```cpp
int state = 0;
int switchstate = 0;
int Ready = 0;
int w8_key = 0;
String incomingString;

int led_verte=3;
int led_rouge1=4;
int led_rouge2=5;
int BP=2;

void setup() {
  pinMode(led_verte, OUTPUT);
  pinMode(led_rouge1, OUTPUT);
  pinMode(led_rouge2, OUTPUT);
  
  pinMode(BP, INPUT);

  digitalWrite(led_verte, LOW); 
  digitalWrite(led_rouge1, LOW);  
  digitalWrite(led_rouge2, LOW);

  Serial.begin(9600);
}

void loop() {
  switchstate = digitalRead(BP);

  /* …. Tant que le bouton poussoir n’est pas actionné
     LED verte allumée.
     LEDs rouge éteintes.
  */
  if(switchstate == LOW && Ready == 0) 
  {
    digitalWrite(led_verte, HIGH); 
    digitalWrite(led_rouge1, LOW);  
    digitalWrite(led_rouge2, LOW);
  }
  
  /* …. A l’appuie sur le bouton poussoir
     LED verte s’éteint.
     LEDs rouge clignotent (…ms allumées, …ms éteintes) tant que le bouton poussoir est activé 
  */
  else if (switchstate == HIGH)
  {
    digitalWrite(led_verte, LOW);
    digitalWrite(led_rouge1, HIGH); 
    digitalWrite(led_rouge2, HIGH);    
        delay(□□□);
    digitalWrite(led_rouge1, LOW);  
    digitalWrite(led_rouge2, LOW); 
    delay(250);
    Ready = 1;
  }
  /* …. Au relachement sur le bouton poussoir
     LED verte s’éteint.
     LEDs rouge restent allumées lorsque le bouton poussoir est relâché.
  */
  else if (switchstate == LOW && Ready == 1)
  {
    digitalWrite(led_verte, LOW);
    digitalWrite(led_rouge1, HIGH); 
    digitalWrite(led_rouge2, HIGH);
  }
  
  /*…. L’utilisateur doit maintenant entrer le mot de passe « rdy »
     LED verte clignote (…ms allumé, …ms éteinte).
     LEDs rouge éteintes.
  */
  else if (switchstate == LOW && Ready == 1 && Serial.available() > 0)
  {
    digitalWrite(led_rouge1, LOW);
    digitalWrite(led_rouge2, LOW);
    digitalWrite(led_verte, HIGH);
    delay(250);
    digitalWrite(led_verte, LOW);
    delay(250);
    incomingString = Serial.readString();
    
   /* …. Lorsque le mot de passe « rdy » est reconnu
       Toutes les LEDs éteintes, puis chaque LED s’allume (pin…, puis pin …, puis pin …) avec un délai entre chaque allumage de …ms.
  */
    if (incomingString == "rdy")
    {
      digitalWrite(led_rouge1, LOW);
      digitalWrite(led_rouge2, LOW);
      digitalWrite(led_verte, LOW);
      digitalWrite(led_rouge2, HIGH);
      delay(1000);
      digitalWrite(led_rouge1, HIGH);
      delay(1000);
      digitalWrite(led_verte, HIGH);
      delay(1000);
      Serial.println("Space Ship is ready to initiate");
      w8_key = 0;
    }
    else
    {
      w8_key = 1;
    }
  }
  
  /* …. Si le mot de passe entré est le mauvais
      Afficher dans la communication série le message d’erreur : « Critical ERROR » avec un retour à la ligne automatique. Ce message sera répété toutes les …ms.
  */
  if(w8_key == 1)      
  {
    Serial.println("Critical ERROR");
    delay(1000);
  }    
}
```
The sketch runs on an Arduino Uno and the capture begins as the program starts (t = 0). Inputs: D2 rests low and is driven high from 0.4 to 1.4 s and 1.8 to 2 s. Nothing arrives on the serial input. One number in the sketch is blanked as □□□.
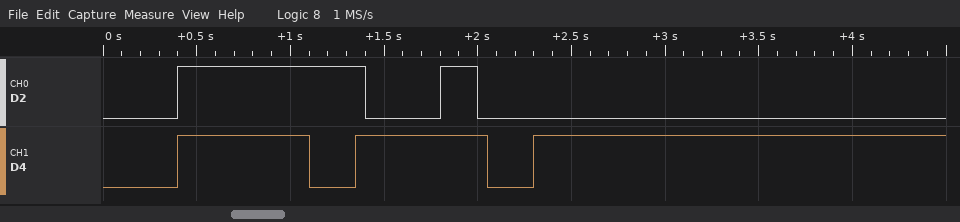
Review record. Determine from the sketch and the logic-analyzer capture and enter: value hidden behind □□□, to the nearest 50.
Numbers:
700
